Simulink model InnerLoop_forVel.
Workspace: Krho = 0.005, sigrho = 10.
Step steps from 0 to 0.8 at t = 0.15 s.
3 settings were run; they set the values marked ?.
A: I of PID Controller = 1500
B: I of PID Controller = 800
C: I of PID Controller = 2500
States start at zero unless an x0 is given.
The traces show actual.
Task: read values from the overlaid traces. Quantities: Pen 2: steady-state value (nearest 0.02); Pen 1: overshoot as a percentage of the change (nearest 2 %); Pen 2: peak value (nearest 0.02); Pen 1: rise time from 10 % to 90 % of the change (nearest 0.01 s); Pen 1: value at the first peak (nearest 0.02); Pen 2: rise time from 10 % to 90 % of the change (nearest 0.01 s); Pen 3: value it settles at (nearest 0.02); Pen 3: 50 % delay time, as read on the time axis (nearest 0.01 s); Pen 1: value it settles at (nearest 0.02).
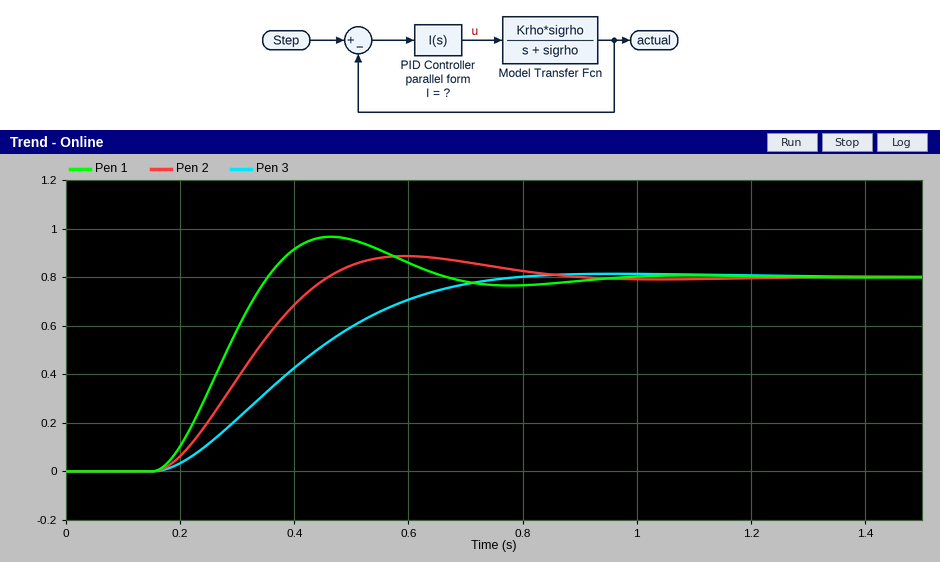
0.80
20 %
0.88
0.14 s
0.96
0.21 s
0.80
0.39 s
0.80
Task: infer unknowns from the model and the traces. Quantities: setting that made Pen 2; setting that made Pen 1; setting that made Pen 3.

A
C
B
